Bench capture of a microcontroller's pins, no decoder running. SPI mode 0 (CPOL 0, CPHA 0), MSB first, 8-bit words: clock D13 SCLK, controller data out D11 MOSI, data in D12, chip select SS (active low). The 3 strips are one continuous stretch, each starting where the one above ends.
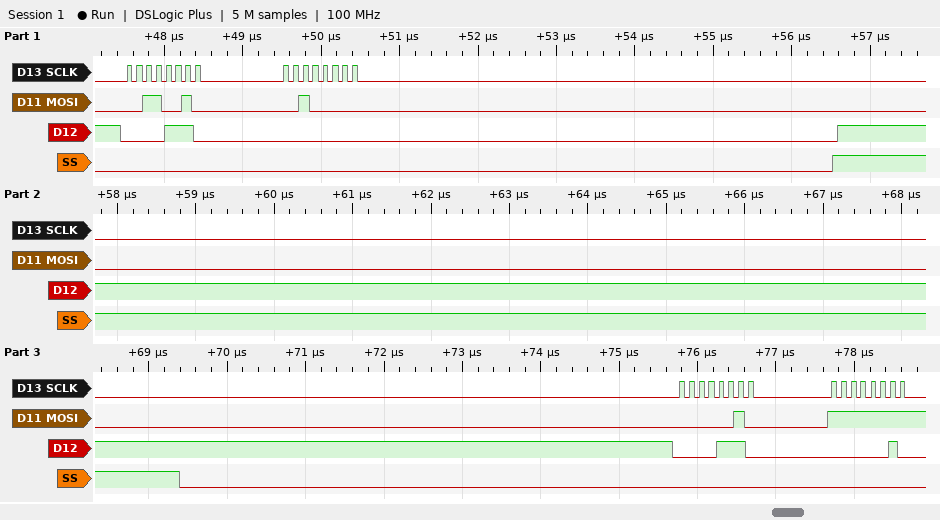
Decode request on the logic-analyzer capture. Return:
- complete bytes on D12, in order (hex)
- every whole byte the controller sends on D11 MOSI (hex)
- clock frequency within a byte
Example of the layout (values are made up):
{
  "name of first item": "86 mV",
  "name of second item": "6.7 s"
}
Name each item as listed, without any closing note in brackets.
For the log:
{
  "complete bytes on D12, in order": "0E 00 0E 02",
  "every whole byte the controller sends on D11 MOSI": "32 20 02 FF",
  "clock frequency within a byte": "8 MHz"
}
